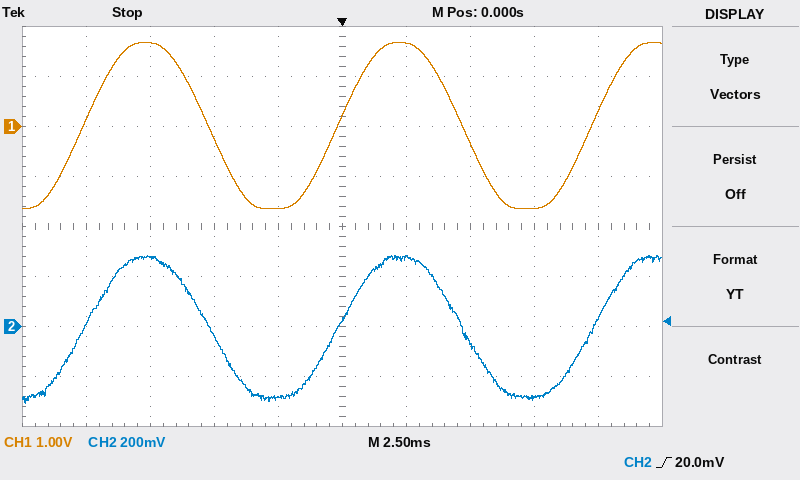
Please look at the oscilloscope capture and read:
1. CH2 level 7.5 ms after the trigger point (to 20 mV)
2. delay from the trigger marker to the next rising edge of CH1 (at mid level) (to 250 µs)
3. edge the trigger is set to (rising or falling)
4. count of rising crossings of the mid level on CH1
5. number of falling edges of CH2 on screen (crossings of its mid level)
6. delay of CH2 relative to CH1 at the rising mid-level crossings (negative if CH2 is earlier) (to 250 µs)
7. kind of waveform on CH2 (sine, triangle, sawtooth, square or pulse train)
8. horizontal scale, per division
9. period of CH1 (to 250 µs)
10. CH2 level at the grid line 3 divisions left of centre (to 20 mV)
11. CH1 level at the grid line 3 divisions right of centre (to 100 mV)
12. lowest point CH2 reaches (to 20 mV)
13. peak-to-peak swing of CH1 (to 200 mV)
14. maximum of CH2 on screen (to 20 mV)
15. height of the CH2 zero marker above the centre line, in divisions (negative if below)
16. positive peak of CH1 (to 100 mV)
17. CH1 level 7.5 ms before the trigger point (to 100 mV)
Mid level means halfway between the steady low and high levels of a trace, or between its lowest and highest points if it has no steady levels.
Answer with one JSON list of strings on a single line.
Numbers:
["-280 mV", "9.75 ms", "rising", "3", "2", "0.00 ms", "sine", "2.5 ms", "10.00 ms", "280 mV", "-1.6 V", "-300 mV", "3.4 V", "280 mV", "-2.0 div", "1.7 V", "1.7 V"]
